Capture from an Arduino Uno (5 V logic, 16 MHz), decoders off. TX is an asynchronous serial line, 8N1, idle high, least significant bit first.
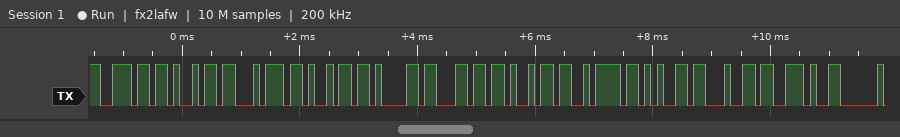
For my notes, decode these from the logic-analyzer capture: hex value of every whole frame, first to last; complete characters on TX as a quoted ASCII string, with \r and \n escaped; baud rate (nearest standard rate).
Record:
0x6E 0x69 0x74 0x69 0x61 0x6C 0x69 0x7A 0x65 0x64 0x2E
"nitialized."
9600 baud
